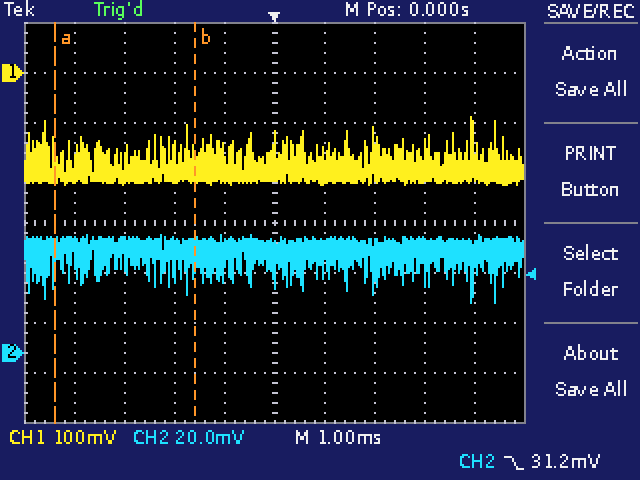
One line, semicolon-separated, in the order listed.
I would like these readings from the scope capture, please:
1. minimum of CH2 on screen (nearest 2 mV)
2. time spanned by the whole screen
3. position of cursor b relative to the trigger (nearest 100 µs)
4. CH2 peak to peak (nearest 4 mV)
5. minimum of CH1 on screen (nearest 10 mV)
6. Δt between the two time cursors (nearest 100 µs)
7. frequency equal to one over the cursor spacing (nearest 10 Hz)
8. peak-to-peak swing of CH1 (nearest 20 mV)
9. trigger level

20 mV; 10 ms; -1.6 ms; 28 mV; -220 mV; 2.8 ms; 360 Hz; 140 mV; 31.2 mV
